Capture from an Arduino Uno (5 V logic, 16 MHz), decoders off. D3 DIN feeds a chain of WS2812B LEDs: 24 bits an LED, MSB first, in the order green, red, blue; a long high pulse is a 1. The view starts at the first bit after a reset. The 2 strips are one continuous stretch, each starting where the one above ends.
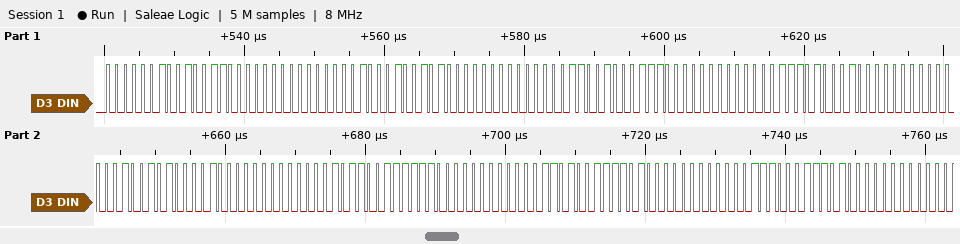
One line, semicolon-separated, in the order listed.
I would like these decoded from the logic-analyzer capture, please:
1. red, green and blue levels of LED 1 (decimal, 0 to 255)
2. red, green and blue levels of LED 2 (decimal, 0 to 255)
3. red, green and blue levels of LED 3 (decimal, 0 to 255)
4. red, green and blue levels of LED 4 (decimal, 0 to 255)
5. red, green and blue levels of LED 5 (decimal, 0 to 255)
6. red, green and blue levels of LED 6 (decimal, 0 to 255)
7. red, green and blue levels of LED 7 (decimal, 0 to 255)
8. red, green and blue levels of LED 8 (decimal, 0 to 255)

76, 2, 0; 74, 4, 0; 71, 6, 0; 68, 7, 0; 66, 9, 0; 63, 11, 0; 61, 13, 0; 58, 14, 0
